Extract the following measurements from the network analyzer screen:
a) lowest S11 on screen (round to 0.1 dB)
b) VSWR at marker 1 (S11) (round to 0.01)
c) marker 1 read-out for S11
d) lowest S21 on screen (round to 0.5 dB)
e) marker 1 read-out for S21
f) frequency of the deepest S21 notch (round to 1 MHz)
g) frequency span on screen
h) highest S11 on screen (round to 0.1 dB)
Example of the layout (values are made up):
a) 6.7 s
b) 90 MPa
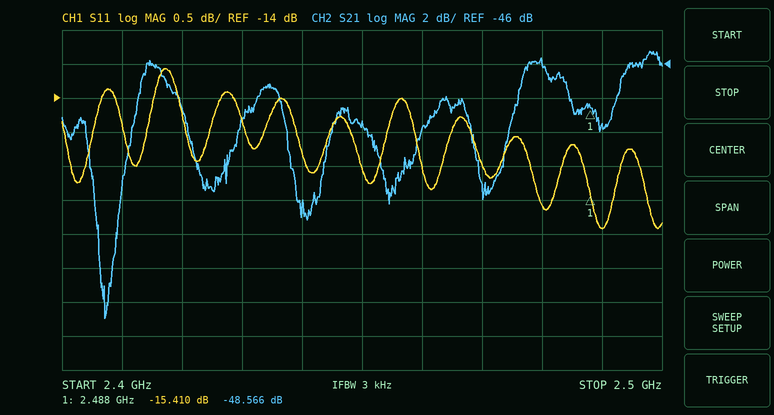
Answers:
a) -15.9 dB
b) 1.41
c) -15.410 dB
d) -61.0 dB
e) -48.566 dB
f) 2.407 GHz
g) 100 MHz
h) -13.6 dB
